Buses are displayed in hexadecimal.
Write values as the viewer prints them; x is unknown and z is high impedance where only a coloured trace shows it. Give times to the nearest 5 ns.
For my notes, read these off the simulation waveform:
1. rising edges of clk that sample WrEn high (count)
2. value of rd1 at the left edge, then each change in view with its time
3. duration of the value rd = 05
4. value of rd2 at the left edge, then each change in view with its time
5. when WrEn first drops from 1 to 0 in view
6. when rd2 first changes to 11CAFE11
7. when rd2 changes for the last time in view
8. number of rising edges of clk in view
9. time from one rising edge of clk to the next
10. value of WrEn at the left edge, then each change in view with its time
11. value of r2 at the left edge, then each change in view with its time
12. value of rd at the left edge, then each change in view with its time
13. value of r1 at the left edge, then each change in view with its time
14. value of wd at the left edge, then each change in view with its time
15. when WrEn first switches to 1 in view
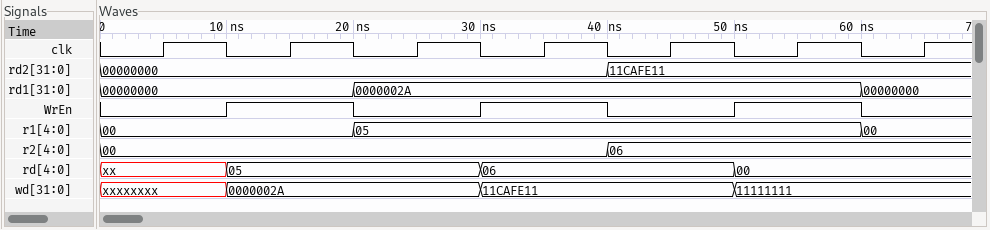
3
00000000, 0000002A at 20 ns, 00000000 at 60 ns
20 ns
00000000, 11CAFE11 at 40 ns
20 ns
40 ns
40 ns
7
10 ns
0, 1 at 10 ns, 0 at 20 ns, 1 at 30 ns, 0 at 40 ns, 1 at 50 ns, 0 at 60 ns
00, 06 at 40 ns
xx, 05 at 10 ns, 06 at 30 ns, 00 at 50 ns
00, 05 at 20 ns, 00 at 60 ns
xxxxxxxx, 0000002A at 10 ns, 11CAFE11 at 30 ns, 11111111 at 50 ns
10 ns
